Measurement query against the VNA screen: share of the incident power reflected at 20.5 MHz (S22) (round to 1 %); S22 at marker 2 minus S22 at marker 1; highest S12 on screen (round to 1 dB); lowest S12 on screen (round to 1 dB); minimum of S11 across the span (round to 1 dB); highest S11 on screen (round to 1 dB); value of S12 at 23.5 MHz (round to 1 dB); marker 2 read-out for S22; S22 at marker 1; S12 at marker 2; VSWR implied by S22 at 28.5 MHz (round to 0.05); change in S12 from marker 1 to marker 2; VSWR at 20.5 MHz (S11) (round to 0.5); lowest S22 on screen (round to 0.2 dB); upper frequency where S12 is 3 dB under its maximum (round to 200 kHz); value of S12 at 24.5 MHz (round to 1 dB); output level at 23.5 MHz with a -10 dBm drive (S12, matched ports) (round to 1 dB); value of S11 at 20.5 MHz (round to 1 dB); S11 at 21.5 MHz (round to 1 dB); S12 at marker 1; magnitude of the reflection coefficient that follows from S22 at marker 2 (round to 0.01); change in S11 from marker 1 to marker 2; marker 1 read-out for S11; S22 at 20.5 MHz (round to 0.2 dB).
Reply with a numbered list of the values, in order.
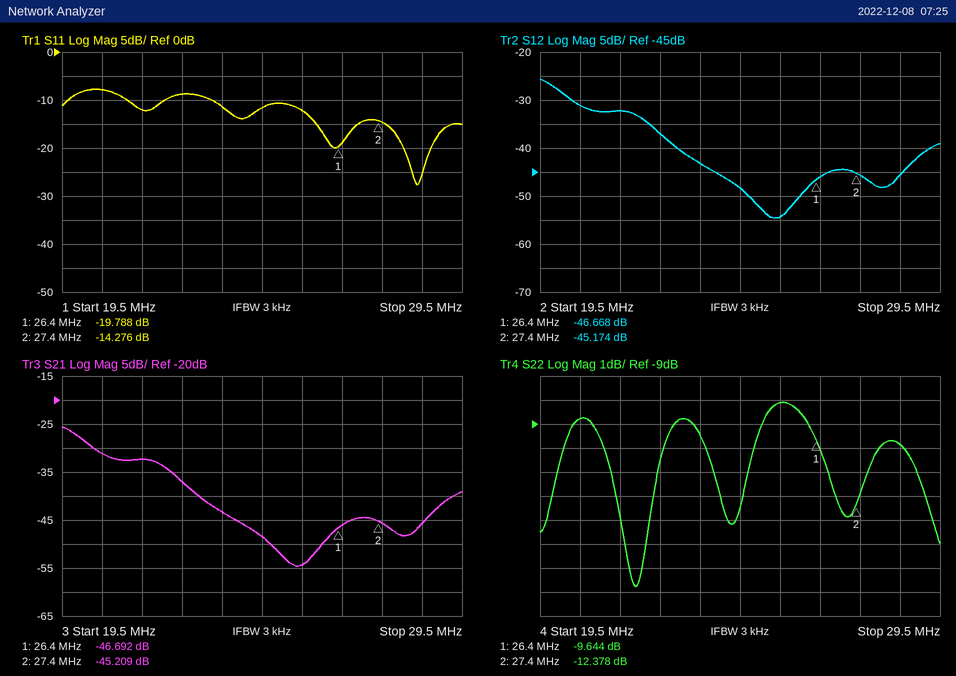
1. 13 %
2. -2.734 dB
3. -26 dB
4. -55 dB
5. -28 dB
6. -8 dB
7. -43 dB
8. -12.378 dB
9. -9.644 dB
10. -45.174 dB
11. 1.95
12. 1.494 dB
13. 2.5
14. -15.8 dB
15. 20.0 MHz
16. -48 dB
17. -53 dBm
18. -8 dB
19. -12 dB
20. -46.668 dB
21. 0.24
22. 5.512 dB
23. -19.788 dB
24. -8.8 dB
